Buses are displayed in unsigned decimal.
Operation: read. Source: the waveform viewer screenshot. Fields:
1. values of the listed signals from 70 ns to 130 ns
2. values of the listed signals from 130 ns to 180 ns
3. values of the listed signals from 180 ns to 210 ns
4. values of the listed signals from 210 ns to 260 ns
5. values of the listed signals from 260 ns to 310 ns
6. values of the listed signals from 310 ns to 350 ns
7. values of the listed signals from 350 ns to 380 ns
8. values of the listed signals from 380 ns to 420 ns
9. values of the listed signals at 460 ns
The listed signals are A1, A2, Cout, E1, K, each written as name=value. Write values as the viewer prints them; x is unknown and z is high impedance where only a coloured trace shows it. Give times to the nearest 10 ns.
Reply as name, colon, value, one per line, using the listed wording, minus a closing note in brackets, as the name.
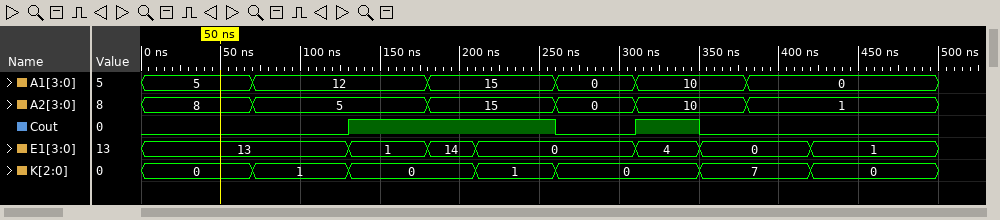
values of the listed signals from 70 ns to 130 ns: A1=12, A2=5, Cout=0, E1=13, K=1
values of the listed signals from 130 ns to 180 ns: A1=12, A2=5, Cout=1, E1=1, K=0
values of the listed signals from 180 ns to 210 ns: A1=15, A2=15, Cout=1, E1=14, K=0
values of the listed signals from 210 ns to 260 ns: A1=15, A2=15, Cout=1, E1=0, K=1
values of the listed signals from 260 ns to 310 ns: A1=0, A2=0, Cout=0, E1=0, K=0
values of the listed signals from 310 ns to 350 ns: A1=10, A2=10, Cout=1, E1=4, K=0
values of the listed signals from 350 ns to 380 ns: A1=10, A2=10, Cout=0, E1=0, K=7
values of the listed signals from 380 ns to 420 ns: A1=0, A2=1, Cout=0, E1=0, K=7
values of the listed signals at 460 ns: A1=0, A2=1, Cout=0, E1=1, K=0
